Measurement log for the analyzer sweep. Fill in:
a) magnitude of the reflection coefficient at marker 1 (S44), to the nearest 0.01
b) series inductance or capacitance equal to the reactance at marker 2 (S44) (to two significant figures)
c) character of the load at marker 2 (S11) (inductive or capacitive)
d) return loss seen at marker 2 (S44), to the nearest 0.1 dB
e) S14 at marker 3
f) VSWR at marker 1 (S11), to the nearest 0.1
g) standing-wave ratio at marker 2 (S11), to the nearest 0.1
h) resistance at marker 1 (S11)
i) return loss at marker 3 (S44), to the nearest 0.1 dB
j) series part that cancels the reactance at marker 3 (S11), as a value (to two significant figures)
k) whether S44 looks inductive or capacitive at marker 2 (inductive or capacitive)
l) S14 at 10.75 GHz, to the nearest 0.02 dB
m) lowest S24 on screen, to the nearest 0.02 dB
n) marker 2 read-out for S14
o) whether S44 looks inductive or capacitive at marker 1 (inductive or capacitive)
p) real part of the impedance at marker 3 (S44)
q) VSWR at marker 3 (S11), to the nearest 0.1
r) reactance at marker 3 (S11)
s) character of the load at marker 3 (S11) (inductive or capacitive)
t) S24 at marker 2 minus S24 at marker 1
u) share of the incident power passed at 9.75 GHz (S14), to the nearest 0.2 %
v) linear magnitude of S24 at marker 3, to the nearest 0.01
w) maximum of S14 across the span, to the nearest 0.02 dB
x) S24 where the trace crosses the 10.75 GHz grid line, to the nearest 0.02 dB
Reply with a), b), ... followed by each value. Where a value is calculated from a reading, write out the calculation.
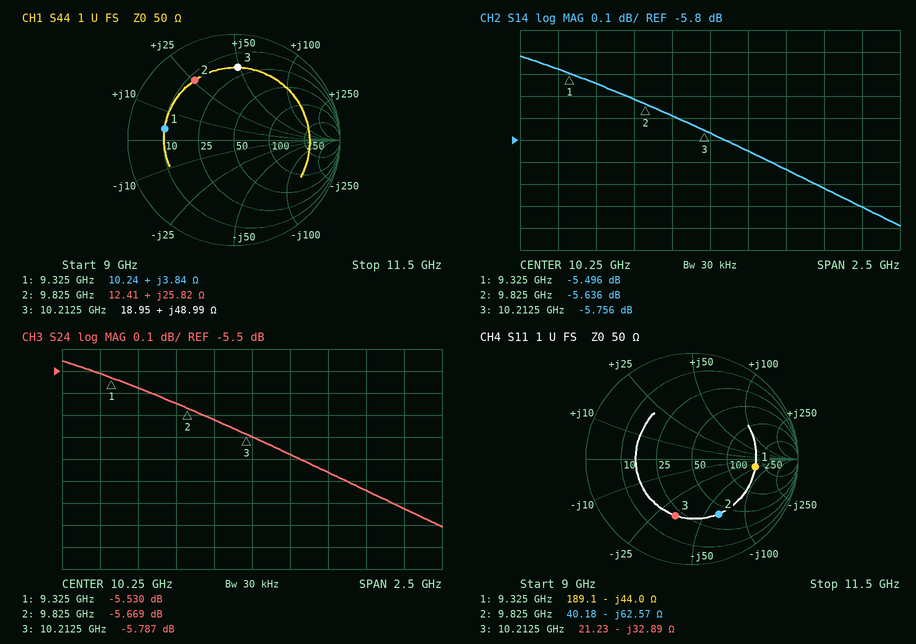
a) 0.66
b) L = 25.82 Ω/(2π × 9.825 GHz) ≈ 418 pH, so 420 pH to two significant figures
c) capacitive
d) 3.4 dB
e) -5.756 dB
f) 4.0
g) 3.7
h) 189.1 Ω
i) 3.3 dB
j) L = 32.89 Ω/(2π × 10.2125 GHz) ≈ 513 pH, so 510 pH to two significant figures
k) inductive
l) -5.94 dB
m) -6.20 dB
n) -5.636 dB
o) inductive
p) 18.95 Ω
q) 3.5
r) -32.89 Ω
s) capacitive
t) -5.669 − (-5.53) = -0.139 dB
u) 10^(-5.62/10) ≈ 27.4 %
v) 10^(-5.787/20) ≈ 0.51
w) -5.42 dB
x) -5.96 dB
